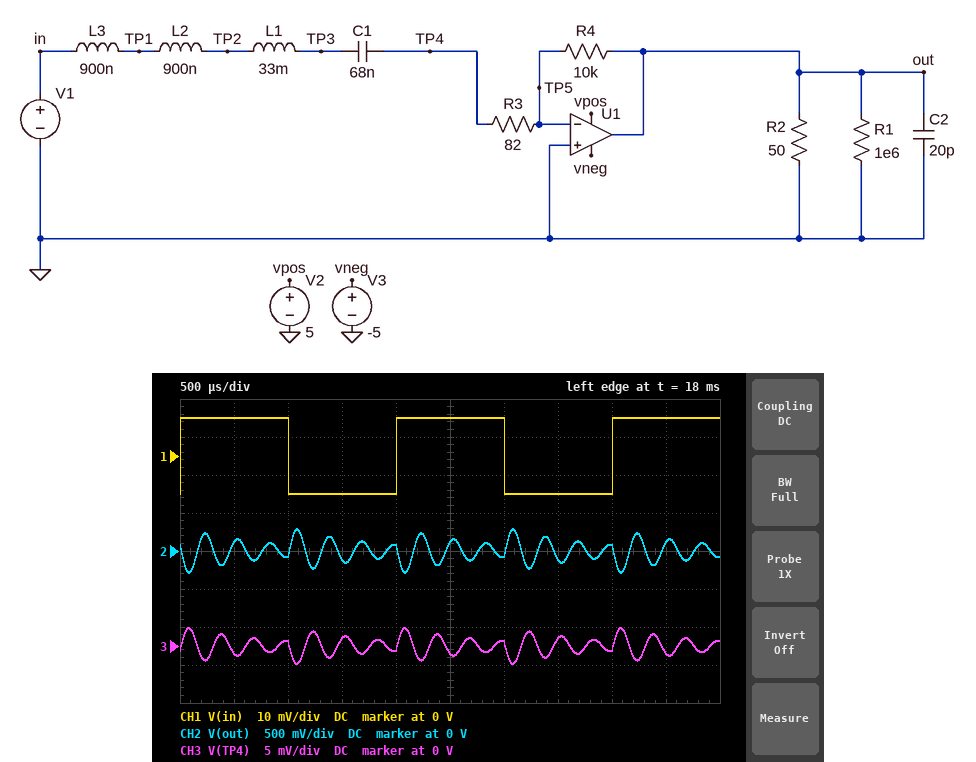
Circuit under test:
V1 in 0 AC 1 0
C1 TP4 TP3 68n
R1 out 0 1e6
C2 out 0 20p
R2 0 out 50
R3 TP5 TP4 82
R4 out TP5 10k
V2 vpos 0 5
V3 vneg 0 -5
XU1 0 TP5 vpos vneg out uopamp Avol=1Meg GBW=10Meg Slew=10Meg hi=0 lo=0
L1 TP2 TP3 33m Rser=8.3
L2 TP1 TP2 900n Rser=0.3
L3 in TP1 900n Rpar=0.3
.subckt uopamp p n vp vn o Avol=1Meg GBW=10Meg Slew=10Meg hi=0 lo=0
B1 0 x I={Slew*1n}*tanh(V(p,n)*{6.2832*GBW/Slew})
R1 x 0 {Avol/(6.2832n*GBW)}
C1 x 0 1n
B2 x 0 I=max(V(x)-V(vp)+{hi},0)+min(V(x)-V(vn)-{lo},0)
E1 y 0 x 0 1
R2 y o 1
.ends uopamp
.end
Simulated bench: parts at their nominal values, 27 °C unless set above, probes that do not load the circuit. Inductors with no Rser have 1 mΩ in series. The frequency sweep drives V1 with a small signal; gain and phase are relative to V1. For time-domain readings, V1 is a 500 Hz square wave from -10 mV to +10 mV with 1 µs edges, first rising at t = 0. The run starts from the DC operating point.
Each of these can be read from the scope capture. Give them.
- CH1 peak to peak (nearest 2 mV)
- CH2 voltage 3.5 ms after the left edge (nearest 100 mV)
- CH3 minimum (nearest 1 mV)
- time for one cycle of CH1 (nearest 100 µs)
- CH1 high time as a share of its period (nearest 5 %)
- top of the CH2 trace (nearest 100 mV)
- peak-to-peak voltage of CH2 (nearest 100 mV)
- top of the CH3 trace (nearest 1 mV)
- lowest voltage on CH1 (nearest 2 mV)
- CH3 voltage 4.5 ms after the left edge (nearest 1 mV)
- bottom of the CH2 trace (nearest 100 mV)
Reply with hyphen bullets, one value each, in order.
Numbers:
- 20 mV
- -100 mV
- -2 mV
- 2.0 ms
- 50 %
- 300 mV
- 600 mV
- 2 mV
- -10 mV
- -1 mV
- -300 mV
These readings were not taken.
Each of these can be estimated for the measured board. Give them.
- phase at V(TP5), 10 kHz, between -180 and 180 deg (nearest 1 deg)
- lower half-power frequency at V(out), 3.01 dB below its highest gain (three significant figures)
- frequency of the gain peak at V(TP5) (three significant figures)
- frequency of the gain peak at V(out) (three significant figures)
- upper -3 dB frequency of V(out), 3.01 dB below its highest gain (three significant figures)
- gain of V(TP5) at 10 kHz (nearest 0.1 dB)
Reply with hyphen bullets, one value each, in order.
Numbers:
- 3 deg
- 3.14 kHz
- 3.37 kHz
- 3.35 kHz
- 3.58 kHz
- -45.2 dB
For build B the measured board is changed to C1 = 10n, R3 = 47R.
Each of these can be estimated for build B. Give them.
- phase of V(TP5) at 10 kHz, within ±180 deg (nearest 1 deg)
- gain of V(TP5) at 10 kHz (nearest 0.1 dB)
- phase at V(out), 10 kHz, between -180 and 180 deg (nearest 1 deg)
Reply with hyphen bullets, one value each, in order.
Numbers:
- 6 deg
- -33.7 dB
- 96 deg
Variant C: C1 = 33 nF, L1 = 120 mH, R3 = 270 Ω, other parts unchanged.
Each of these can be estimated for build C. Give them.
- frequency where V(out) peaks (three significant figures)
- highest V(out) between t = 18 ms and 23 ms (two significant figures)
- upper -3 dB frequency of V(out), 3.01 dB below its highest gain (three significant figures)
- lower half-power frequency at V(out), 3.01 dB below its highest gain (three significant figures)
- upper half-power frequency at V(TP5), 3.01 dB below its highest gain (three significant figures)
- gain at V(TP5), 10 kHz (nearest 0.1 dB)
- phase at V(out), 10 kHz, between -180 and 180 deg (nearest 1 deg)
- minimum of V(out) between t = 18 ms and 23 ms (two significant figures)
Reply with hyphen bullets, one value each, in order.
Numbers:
- 2.53 kHz
- 140 mV
- 2.72 kHz
- 2.35 kHz
- 2.75 kHz
- -56.8 dB
- 92 deg
- -140 mV
